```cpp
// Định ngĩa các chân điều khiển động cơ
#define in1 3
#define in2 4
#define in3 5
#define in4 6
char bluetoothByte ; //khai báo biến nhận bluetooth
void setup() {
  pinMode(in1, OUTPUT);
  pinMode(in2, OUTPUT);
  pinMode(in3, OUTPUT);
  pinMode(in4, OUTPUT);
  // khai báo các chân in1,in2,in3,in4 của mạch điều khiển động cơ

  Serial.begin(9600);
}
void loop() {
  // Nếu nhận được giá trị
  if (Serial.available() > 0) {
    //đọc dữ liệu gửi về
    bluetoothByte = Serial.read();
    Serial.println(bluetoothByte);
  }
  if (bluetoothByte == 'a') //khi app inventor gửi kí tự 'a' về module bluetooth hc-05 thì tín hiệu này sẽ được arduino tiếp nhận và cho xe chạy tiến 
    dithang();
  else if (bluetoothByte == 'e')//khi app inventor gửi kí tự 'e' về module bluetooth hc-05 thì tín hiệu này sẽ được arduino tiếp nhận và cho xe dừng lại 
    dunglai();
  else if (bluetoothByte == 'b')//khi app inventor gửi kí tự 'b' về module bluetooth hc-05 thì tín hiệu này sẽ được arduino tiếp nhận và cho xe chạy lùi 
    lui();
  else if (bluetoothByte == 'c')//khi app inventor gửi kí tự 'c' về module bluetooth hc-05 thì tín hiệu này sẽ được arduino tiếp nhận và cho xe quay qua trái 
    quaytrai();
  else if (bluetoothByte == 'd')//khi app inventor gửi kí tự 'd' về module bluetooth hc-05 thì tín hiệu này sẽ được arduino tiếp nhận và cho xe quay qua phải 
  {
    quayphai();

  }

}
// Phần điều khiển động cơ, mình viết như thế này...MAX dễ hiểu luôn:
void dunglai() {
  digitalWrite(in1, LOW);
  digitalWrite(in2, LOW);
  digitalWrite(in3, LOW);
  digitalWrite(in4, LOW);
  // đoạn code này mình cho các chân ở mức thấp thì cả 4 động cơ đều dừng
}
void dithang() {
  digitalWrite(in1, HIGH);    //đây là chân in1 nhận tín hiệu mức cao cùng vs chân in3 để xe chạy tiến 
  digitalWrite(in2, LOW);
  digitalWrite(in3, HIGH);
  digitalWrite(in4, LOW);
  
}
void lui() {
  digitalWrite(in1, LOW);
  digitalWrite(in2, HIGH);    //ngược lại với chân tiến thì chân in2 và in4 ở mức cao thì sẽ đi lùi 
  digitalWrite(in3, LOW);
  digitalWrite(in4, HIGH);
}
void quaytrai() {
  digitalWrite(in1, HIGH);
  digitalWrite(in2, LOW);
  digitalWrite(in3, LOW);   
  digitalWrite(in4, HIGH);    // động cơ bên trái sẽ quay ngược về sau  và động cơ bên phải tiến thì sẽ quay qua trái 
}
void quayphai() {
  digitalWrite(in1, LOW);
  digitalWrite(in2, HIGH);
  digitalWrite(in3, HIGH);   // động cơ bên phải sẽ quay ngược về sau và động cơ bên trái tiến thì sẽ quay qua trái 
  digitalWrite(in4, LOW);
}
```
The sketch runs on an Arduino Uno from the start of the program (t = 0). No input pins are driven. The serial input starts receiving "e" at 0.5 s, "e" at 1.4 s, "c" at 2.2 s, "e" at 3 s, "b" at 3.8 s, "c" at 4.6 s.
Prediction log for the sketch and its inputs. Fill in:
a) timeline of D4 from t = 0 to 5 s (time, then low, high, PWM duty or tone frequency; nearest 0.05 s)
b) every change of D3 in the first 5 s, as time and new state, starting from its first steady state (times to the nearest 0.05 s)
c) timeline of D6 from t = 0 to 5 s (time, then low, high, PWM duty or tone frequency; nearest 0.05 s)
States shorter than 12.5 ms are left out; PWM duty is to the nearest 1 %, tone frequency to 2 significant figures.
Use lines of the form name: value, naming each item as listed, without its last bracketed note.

timeline of D4 from t = 0 to 5 s: 0 s low; 3.8 s high; 4.6 s low
every change of D3 in the first 5 s, as time and new state, starting from its first steady state: 0 s low; 2.2 s high; 3 s low; 4.6 s high
timeline of D6 from t = 0 to 5 s: 0 s low; 2.2 s high; 3 s low; 3.8 s high
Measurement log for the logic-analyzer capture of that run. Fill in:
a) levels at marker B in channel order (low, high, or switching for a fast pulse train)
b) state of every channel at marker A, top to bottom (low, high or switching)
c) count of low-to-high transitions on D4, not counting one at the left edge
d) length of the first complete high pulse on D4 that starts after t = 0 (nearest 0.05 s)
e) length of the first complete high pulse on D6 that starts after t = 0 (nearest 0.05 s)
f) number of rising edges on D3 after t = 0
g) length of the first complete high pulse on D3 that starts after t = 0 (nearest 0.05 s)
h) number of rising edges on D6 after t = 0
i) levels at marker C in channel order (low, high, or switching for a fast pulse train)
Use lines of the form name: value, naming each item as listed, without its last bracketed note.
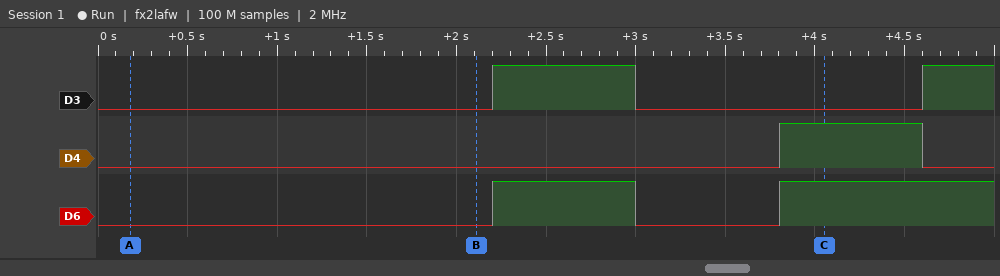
levels at marker B in channel order: D3 low, D4 low, D6 low
state of every channel at marker A, top to bottom: D3 low, D4 low, D6 low
count of low-to-high transitions on D4, not counting one at the left edge: 1
length of the first complete high pulse on D4 that starts after t = 0: 0.80 s
length of the first complete high pulse on D6 that starts after t = 0: 0.80 s
number of rising edges on D3 after t = 0: 2
length of the first complete high pulse on D3 that starts after t = 0: 0.80 s
number of rising edges on D6 after t = 0: 2
levels at marker C in channel order: D3 low, D4 high, D6 high
